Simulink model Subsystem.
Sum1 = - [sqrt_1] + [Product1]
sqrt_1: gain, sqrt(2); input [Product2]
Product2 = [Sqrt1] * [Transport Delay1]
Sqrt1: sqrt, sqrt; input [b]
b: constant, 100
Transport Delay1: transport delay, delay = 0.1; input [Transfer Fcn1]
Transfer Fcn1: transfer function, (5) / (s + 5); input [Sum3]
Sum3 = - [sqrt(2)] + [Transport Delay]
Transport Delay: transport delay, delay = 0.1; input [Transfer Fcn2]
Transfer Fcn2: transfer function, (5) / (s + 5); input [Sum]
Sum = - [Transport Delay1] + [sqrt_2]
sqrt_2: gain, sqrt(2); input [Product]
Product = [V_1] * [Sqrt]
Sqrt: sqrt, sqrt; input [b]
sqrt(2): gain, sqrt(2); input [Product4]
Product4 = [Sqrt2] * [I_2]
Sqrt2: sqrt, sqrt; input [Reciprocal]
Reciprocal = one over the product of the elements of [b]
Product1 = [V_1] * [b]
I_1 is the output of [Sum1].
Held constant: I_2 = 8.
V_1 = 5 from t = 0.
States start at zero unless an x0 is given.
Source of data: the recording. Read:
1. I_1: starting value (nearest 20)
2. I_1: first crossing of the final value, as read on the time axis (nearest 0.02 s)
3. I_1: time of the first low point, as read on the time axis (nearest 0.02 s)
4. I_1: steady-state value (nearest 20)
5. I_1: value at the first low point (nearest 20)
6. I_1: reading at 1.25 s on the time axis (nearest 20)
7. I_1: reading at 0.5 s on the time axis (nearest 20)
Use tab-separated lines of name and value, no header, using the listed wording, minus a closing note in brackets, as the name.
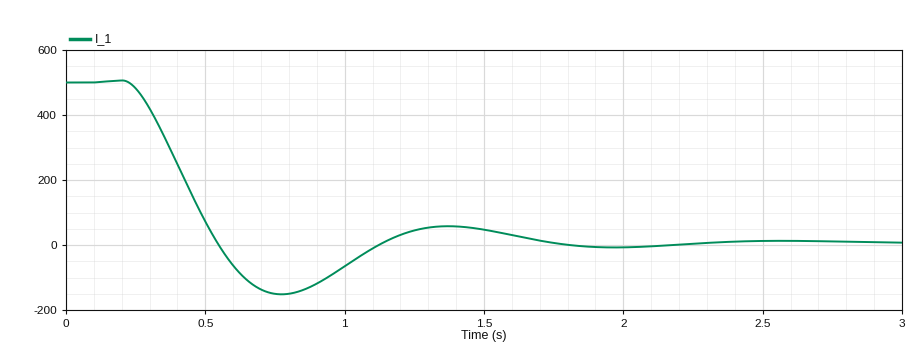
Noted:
I_1: starting value	500
I_1: first crossing of the final value, as read on the time axis	0.54 s
I_1: time of the first low point, as read on the time axis	0.78 s
I_1: steady-state value	0
I_1: value at the first low point	-160
I_1: reading at 1.25 s on the time axis	40
I_1: reading at 0.5 s on the time axis	80
